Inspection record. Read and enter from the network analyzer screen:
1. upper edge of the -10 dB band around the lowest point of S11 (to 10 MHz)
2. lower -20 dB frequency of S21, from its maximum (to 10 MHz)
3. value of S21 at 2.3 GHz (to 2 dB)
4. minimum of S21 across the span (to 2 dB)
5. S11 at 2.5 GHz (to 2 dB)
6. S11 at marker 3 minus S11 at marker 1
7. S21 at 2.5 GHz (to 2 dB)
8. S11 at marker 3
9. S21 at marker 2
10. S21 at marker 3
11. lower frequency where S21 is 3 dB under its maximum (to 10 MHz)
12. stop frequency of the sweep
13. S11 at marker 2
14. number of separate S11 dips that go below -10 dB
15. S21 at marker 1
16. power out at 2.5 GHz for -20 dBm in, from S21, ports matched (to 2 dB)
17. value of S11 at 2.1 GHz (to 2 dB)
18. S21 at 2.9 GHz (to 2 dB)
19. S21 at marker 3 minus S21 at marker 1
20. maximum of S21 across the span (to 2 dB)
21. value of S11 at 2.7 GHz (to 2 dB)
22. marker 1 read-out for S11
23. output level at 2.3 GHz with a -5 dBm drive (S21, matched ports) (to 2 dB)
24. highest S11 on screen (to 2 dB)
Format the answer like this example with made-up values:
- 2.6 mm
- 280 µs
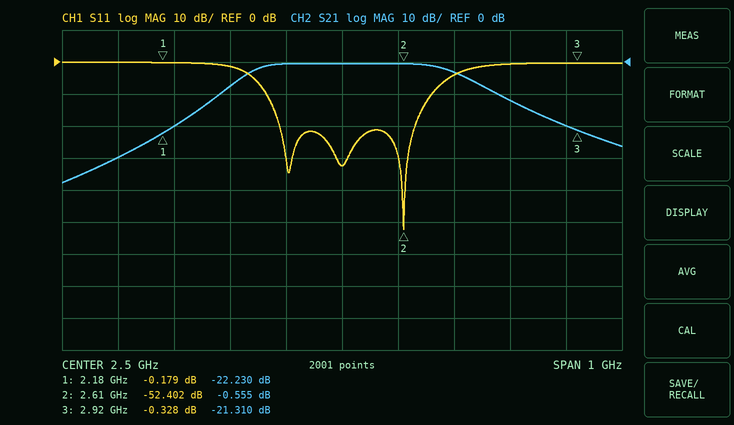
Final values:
- 2.66 GHz
- 2.20 GHz
- -8 dB
- -38 dB
- -32 dB
- -0.149 dB
- 0 dB
- -0.328 dB
- -0.555 dB
- -21.310 dB
- 2.33 GHz
- 3 GHz
- -52.402 dB
- 3
- -22.230 dB
- -20 dBm
- 0 dB
- -20 dB
- 0.920 dB
- 0 dB
- -4 dB
- -0.179 dB
- -12 dBm
- 0 dB
